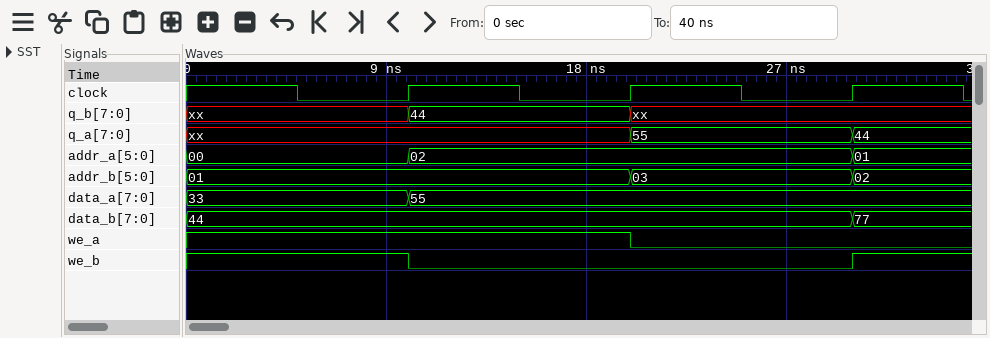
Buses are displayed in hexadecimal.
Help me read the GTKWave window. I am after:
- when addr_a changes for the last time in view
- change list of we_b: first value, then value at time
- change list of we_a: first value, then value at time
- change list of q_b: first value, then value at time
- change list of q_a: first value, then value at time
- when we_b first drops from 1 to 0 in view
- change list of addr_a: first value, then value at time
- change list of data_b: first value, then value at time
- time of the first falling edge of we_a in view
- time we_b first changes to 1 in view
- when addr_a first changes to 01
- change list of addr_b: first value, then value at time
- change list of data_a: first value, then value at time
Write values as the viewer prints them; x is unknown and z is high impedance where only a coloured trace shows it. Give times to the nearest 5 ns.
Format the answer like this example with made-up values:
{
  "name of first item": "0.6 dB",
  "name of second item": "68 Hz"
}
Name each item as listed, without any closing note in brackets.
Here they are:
{
  "when addr_a changes for the last time in view": "30 ns",
  "change list of we_b: first value, then value at time": "1, 0 at 10 ns, 1 at 30 ns",
  "change list of we_a: first value, then value at time": "1, 0 at 20 ns",
  "change list of q_b: first value, then value at time": "xx, 44 at 10 ns, xx at 20 ns",
  "change list of q_a: first value, then value at time": "xx, 55 at 20 ns, 44 at 30 ns",
  "when we_b first drops from 1 to 0 in view": "10 ns",
  "change list of addr_a: first value, then value at time": "00, 02 at 10 ns, 01 at 30 ns",
  "change list of data_b: first value, then value at time": "44, 77 at 30 ns",
  "time of the first falling edge of we_a in view": "20 ns",
  "time we_b first changes to 1 in view": "30 ns",
  "when addr_a first changes to 01": "30 ns",
  "change list of addr_b: first value, then value at time": "01, 03 at 20 ns, 02 at 30 ns",
  "change list of data_a: first value, then value at time": "33, 55 at 10 ns"
}
